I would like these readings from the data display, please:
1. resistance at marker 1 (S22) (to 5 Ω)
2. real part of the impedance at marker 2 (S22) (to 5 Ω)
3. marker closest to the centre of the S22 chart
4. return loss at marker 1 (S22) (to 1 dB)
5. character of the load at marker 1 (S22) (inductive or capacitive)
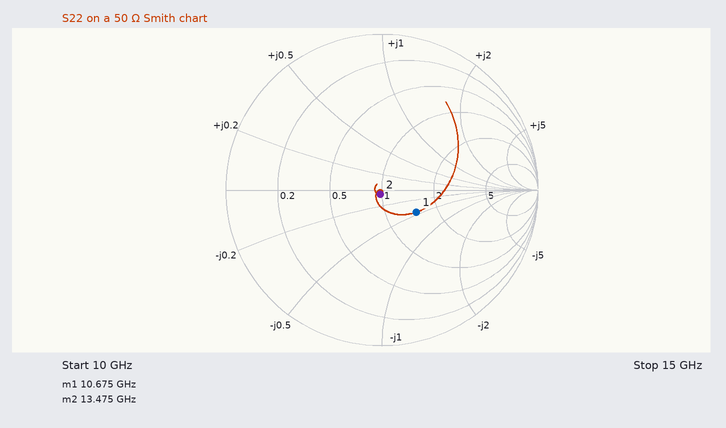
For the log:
75 Ω
50 Ω
marker 2
12 dB
capacitive
